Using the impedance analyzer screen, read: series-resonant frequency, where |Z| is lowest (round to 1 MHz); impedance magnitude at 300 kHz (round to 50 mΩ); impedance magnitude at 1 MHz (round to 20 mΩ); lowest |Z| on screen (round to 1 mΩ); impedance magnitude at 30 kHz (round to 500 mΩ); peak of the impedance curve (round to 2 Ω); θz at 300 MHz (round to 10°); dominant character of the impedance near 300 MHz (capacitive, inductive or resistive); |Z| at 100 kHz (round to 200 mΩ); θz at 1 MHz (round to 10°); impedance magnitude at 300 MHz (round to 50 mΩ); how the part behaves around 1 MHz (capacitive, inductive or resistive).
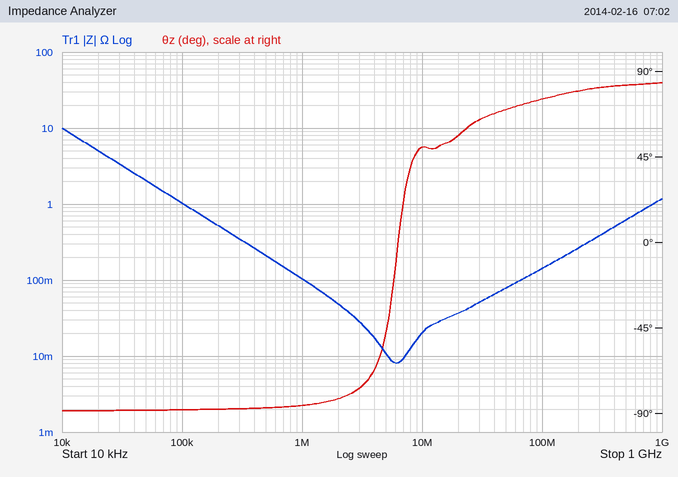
6 MHz
350 mΩ
100 mΩ
8 mΩ
3.5 Ω
10 Ω
80°
inductive
1.0 Ω
-90°
400 mΩ
capacitive
